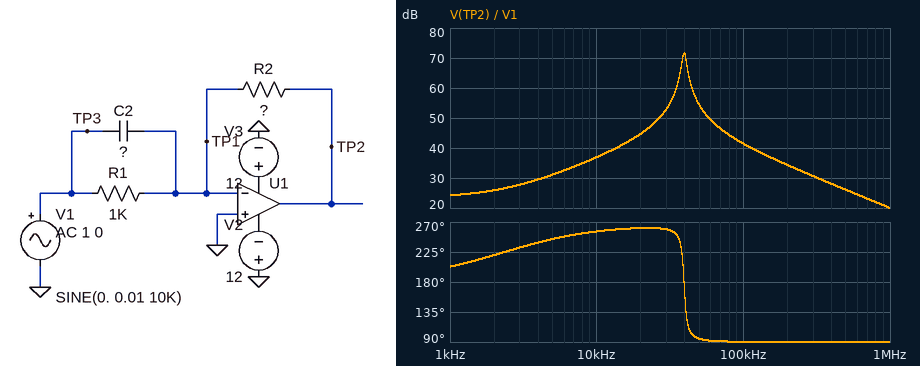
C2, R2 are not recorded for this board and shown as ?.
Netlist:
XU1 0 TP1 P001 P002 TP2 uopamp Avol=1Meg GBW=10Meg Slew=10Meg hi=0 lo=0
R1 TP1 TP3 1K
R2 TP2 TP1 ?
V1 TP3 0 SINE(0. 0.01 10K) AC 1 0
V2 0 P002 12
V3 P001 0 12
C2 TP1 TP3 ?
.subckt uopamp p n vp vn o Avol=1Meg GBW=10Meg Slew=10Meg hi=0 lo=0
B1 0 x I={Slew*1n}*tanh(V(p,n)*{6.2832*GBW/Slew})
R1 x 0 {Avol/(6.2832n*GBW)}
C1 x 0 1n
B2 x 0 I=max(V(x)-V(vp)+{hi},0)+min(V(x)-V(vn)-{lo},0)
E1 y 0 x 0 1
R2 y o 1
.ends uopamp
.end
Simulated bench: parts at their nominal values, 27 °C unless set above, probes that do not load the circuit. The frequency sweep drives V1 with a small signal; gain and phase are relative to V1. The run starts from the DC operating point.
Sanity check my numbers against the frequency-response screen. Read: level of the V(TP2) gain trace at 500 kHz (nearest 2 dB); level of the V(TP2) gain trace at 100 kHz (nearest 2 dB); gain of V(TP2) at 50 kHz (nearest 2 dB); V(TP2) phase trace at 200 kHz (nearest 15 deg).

26 dB
42 dB
54 dB
90 deg
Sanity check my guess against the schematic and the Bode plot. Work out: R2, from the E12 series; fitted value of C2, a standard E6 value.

15 kΩ
68 nF
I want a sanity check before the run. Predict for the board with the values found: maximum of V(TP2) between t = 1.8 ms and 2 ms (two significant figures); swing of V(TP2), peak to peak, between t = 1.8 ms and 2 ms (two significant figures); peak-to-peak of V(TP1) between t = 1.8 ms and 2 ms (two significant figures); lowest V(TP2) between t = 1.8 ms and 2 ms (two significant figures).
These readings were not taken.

700 mV
1.4 V
1.4 mV
-700 mV
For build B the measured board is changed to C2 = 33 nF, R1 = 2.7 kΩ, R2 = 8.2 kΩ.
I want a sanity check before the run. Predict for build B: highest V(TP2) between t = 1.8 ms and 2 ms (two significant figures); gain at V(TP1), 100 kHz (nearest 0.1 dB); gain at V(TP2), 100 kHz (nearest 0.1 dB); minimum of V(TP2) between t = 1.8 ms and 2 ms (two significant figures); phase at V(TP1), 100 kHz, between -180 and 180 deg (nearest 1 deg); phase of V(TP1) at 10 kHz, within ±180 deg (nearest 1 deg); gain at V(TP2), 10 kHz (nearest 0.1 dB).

180 mV
7.7 dB
47.7 dB
-180 mV
2 deg
170 deg
24.9 dB
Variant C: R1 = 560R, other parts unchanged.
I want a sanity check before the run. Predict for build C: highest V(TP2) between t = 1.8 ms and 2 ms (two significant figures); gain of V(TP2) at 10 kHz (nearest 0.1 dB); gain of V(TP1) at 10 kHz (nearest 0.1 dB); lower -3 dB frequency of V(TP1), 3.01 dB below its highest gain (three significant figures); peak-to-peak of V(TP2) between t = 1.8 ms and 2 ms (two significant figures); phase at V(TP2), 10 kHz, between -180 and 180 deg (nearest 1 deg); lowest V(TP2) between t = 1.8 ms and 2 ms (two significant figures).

740 mV
37.4 dB
-22.6 dB
37.6 kHz
1.5 V
-114 deg
-740 mV
